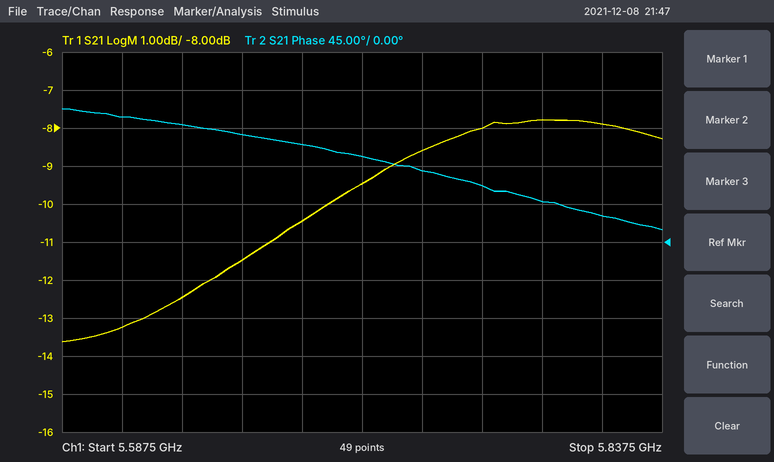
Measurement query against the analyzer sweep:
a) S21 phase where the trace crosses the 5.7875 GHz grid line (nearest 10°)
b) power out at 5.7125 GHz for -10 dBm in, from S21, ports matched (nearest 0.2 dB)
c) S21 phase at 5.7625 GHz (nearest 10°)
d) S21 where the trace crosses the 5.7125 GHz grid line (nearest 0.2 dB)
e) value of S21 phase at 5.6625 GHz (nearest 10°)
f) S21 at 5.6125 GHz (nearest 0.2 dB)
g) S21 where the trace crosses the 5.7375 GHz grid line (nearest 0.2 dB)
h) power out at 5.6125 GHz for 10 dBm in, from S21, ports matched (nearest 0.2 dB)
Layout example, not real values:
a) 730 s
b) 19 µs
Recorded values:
a) 50°
b) -19.4 dBm
c) 70°
d) -9.4 dB
e) 130°
f) -13.2 dB
g) -8.6 dB
h) -3.2 dBm
